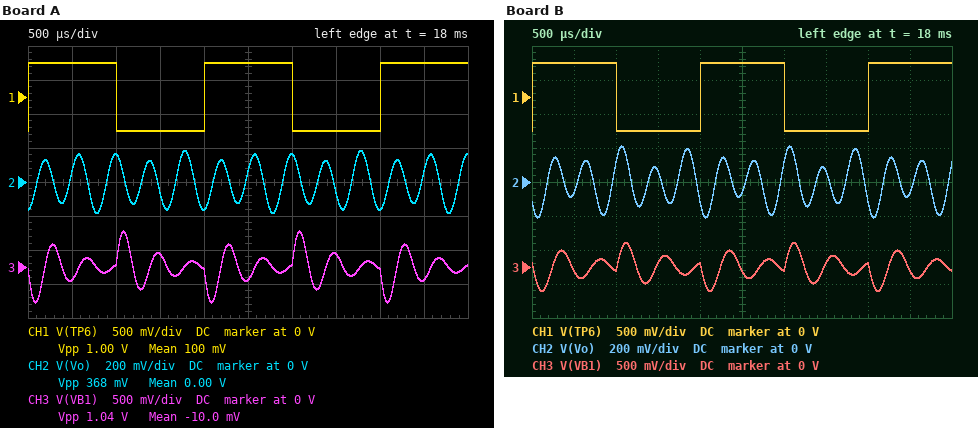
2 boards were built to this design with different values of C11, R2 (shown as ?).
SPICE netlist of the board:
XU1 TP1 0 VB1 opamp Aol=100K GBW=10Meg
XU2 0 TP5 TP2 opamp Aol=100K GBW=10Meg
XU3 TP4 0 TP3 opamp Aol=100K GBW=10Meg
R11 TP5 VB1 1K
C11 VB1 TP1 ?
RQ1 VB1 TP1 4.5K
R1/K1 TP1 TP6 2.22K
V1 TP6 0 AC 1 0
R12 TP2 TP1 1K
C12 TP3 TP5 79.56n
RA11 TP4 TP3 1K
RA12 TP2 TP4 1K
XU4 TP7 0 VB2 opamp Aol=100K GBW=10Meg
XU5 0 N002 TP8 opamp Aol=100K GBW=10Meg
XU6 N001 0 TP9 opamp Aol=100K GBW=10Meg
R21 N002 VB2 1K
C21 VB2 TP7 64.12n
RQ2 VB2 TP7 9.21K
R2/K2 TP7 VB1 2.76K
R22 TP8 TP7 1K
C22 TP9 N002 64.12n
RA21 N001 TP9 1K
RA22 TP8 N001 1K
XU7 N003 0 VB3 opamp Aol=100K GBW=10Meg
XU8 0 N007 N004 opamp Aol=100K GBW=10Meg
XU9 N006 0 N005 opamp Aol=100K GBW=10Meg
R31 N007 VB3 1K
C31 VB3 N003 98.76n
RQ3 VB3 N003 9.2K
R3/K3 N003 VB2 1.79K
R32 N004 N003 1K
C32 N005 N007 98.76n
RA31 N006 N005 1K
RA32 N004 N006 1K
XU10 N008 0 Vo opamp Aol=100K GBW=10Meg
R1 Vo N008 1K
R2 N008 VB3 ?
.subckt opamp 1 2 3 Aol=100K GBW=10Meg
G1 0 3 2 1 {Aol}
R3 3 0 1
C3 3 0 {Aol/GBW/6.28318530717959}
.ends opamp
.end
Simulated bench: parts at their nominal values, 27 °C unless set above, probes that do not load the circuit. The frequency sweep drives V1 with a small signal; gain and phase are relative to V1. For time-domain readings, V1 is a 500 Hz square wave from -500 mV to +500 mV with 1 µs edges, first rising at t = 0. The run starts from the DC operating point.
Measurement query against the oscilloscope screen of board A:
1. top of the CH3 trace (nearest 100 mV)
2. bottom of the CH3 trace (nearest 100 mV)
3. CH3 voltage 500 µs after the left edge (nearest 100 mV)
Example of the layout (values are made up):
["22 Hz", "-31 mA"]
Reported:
["500 mV", "-500 mV", "-200 mV"]
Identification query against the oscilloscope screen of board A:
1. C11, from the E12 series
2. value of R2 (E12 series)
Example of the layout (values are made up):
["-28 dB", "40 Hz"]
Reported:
["47 nF", "3.3 kΩ"]
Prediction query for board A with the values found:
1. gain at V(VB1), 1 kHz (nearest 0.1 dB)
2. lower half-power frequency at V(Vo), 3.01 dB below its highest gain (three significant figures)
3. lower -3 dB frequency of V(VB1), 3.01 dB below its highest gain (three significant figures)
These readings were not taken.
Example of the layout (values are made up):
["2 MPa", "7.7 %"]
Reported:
["-11.6 dB", "2.35 kHz", "2.25 kHz"]
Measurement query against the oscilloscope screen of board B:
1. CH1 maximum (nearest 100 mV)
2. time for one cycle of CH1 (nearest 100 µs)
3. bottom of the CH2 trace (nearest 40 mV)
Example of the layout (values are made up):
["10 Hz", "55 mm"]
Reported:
["500 mV", "2.0 ms", "-200 mV"]
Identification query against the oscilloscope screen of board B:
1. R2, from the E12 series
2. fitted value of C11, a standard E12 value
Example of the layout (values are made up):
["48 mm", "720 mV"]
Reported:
["2.2 kΩ", "68 nF"]
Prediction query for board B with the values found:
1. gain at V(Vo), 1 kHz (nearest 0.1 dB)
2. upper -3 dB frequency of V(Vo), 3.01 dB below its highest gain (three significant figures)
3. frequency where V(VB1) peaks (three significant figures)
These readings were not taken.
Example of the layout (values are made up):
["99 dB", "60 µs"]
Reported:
["-38.0 dB", "2.55 kHz", "2.16 kHz"]
